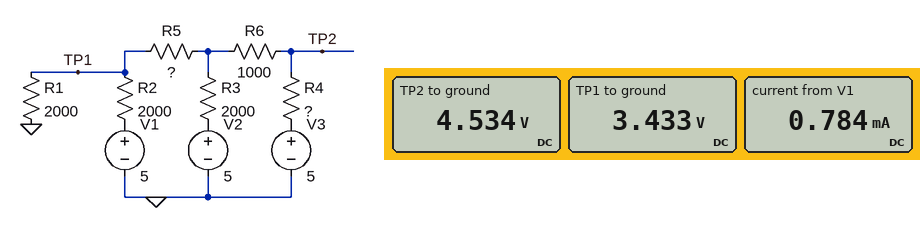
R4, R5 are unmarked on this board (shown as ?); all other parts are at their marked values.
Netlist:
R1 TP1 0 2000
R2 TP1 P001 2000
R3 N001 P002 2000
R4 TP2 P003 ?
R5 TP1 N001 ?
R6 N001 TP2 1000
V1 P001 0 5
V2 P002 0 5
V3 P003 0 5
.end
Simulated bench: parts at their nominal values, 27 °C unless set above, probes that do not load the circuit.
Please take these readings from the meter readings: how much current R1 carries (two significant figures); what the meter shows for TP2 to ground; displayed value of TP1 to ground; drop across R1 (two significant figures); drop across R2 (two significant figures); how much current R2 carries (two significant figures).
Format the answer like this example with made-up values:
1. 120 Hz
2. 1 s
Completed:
1. 1.7 mA
2. 4.534 V
3. 3.433 V
4. 3.4 V
5. 1.6 V
6. 780 µA
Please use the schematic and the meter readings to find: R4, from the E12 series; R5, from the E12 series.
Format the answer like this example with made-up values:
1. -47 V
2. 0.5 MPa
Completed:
1. 1 kΩ
2. 680 Ω
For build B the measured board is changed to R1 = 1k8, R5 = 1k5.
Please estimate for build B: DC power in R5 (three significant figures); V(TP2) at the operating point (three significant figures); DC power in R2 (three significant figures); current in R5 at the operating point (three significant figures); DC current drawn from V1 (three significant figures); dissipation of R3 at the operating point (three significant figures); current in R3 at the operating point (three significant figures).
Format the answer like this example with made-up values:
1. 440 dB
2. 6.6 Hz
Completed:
1. 874 µW
2. 4.62 V
3. 1.82 mW
4. 763 µA
5. 954 µA
6. 291 µW
7. 382 µA
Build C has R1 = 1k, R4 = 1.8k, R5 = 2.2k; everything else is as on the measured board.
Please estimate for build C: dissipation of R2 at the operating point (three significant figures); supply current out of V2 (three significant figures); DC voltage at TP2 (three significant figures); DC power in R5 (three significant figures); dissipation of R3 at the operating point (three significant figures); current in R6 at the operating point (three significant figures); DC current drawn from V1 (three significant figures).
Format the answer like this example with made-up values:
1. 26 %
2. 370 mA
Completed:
1. 3.87 mW
2. 482 µA
3. 4.38 V
4. 1.50 mW
5. 465 µW
6. 344 µA
7. 1.39 mA
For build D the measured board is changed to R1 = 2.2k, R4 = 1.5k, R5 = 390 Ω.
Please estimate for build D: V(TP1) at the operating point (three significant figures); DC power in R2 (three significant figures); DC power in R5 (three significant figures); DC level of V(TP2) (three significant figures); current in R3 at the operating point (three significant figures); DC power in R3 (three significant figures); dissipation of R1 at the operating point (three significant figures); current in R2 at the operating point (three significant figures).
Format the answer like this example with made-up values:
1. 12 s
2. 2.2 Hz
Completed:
1. 3.60 V
2. 983 µW
3. 340 µW
4. 4.38 V
5. 519 µA
6. 539 µW
7. 5.88 mW
8. 701 µA
